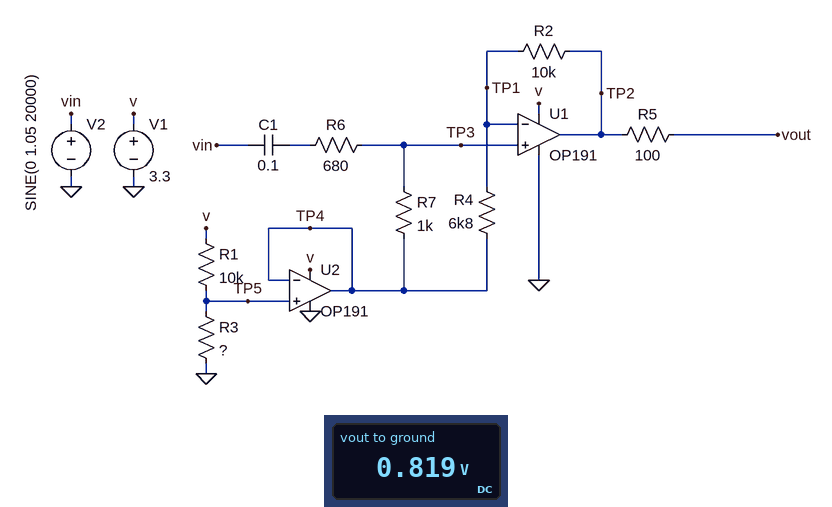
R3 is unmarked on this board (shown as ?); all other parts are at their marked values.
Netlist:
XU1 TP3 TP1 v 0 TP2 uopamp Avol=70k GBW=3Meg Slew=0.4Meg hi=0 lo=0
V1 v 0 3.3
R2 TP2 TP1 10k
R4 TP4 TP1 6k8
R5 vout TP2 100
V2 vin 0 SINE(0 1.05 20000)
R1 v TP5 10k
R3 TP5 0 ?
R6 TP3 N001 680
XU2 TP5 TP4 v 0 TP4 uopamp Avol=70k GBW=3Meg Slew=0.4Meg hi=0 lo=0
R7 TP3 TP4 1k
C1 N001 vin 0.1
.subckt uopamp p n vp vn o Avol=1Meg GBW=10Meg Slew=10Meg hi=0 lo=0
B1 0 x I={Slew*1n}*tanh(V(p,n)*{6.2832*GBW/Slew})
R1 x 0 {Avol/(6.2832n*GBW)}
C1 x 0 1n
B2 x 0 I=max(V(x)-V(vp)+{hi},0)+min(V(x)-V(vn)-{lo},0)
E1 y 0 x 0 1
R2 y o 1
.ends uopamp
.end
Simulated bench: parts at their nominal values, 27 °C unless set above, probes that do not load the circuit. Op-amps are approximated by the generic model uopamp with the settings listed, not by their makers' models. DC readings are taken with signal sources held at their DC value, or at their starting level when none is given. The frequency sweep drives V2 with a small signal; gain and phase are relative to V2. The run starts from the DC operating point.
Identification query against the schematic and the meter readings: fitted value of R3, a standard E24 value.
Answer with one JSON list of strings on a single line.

["3.3 kΩ"]
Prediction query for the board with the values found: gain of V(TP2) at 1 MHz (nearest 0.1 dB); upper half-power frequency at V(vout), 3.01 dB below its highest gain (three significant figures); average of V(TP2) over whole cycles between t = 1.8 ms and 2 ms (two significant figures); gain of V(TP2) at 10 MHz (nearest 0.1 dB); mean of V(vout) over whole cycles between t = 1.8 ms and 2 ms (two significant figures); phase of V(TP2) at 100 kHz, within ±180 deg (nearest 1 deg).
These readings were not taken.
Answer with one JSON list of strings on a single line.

["1.1 dB", "1.21 MHz", "970 mV", "-15.0 dB", "970 mV", "-5 deg"]
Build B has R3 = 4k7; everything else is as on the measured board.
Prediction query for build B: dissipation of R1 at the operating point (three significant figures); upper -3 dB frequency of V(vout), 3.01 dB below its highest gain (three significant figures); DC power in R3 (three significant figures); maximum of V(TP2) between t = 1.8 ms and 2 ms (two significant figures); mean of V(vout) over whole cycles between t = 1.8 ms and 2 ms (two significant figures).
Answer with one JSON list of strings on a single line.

["504 µW", "1.21 MHz", "237 µW", "2.6 V", "1.1 V"]
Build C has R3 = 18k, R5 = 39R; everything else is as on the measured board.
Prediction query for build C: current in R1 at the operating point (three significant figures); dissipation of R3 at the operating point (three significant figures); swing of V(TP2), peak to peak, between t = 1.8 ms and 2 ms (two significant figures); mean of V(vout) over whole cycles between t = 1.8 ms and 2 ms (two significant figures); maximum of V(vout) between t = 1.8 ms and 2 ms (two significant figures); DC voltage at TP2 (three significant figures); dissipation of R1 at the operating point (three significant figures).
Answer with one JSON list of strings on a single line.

["118 µA", "250 µW", "2.7 V", "2.1 V", "3.3 V", "2.12 V", "139 µW"]
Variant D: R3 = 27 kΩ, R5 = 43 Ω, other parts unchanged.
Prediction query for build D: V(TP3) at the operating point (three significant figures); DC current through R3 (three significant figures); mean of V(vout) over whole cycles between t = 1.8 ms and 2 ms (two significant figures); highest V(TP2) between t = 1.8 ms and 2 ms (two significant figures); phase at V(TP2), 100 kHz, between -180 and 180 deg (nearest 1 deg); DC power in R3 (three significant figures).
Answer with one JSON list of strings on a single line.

["2.41 V", "89.2 µA", "2.3 V", "3.3 V", "-5 deg", "215 µW"]
